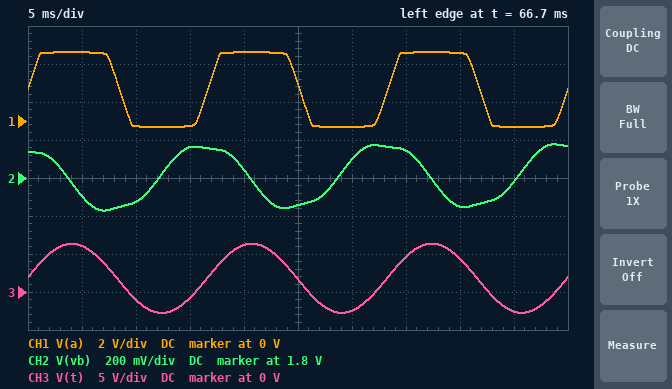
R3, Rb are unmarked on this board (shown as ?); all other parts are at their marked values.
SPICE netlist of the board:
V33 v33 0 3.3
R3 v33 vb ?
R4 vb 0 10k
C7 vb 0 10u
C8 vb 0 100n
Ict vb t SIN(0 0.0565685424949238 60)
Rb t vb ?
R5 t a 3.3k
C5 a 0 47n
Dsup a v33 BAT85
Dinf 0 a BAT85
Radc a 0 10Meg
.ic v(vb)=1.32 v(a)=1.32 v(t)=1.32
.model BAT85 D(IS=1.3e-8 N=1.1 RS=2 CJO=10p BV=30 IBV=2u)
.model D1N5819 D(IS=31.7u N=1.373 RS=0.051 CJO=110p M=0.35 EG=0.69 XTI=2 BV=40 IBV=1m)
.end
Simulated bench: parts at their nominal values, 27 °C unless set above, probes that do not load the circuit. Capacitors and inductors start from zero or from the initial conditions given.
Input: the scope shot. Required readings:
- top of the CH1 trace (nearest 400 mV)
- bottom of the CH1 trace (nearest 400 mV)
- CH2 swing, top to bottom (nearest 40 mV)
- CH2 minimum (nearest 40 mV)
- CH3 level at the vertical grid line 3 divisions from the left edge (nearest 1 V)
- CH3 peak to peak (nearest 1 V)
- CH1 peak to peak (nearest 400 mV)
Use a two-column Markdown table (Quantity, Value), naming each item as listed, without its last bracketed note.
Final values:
| Quantity | Value |
|---|---|
| top of the CH1 trace | 3.6 V |
| bottom of the CH1 trace | -400 mV |
| CH2 swing, top to bottom | 360 mV |
| CH2 minimum | 1.64 V |
| CH3 level at the vertical grid line 3 divisions from the left edge | -1 V |
| CH3 peak to peak | 9 V |
| CH1 peak to peak | 4.0 V |
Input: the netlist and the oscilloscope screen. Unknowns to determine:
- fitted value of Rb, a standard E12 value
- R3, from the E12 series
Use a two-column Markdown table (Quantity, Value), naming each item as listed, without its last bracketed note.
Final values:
| Quantity | Value |
|---|---|
| fitted value of Rb, a standard E12 value | 82 Ω |
| R3, from the E12 series | 6.8 kΩ |
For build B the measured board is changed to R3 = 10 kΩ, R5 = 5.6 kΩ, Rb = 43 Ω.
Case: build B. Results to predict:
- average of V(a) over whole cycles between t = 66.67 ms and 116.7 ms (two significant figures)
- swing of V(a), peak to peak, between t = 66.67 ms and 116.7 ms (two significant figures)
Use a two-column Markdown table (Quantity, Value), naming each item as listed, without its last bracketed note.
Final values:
| Quantity | Value |
|---|---|
| average of V(a) over whole cycles between t = 66.67 ms and 116.7 ms | 1.6 V |
| swing of V(a), peak to peak, between t = 66.67 ms and 116.7 ms | 3.8 V |
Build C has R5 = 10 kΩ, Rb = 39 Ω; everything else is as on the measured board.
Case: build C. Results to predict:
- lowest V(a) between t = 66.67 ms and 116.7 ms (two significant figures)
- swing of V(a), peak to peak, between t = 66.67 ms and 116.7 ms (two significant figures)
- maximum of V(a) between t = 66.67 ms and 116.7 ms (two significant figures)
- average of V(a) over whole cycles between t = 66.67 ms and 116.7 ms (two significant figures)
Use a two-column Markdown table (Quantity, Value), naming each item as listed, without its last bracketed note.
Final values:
| Quantity | Value |
|---|---|
| lowest V(a) between t = 66.67 ms and 116.7 ms | -200 mV |
| swing of V(a), peak to peak, between t = 66.67 ms and 116.7 ms | 3.7 V |
| maximum of V(a) between t = 66.67 ms and 116.7 ms | 3.5 V |
| average of V(a) over whole cycles between t = 66.67 ms and 116.7 ms | 1.8 V |
